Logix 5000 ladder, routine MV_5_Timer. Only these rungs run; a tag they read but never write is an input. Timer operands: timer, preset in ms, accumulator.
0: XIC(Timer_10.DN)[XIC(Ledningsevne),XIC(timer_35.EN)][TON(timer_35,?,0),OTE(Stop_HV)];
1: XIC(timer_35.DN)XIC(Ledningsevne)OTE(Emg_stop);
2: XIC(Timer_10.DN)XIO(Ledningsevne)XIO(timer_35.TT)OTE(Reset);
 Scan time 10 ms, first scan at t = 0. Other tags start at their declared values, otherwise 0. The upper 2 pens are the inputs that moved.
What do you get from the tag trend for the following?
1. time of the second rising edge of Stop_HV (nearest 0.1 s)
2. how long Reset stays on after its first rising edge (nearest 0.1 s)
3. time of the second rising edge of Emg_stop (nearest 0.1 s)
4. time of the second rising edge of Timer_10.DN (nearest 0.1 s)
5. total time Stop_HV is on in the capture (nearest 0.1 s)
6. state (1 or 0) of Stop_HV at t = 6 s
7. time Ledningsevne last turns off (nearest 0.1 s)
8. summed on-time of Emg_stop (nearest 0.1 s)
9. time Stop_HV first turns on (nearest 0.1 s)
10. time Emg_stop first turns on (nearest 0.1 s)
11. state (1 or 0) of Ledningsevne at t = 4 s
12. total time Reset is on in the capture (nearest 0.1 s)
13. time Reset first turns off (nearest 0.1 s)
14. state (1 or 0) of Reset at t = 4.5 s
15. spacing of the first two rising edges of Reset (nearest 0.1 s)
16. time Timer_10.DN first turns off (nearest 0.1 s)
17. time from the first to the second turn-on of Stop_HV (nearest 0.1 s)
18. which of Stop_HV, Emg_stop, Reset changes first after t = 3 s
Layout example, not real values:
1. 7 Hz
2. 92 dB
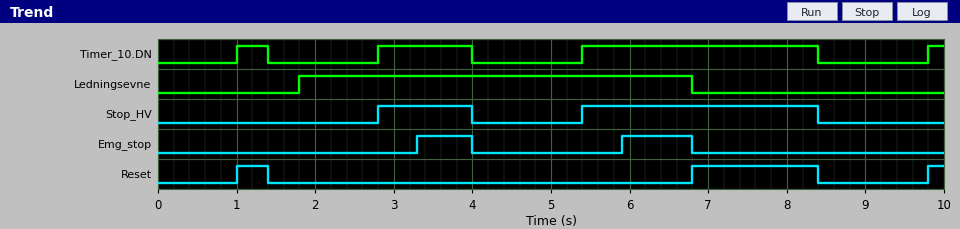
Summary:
1. 5.4 s
2. 0.4 s
3. 5.9 s
4. 2.8 s
5. 4.2 s
6. 1
7. 6.8 s
8. 1.6 s
9. 2.8 s
10. 3.3 s
11. 1
12. 2.2 s
13. 1.4 s
14. 0
15. 5.8 s
16. 1.4 s
17. 2.6 s
18. Emg_stop
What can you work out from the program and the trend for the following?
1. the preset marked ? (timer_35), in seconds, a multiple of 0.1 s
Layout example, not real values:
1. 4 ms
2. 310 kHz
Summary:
1. 0.5 s
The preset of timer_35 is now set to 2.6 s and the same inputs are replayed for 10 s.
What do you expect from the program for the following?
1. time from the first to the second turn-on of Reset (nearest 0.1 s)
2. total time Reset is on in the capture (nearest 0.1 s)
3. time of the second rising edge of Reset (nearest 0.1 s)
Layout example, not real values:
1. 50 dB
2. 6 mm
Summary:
1. 7.0 s
2. 1.0 s
3. 8.0 s
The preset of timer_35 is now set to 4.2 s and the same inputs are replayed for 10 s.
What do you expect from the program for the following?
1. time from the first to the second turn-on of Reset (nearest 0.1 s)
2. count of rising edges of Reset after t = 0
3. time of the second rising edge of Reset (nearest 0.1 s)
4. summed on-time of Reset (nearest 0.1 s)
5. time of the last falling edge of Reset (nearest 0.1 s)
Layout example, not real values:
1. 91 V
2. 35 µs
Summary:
1. 8.8 s
2. 2
3. 9.8 s
4. 0.6 s
5. 1.4 s
